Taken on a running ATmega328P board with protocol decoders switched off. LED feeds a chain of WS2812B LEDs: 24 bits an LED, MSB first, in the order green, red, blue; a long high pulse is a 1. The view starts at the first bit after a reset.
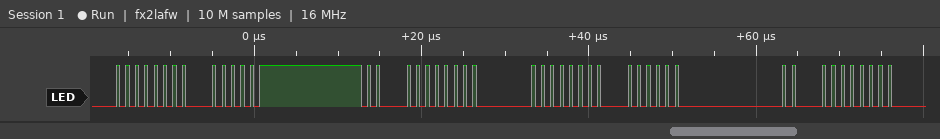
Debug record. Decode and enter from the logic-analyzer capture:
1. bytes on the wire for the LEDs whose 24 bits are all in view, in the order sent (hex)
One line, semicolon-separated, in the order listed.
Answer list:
00 04 00 00 00 00
